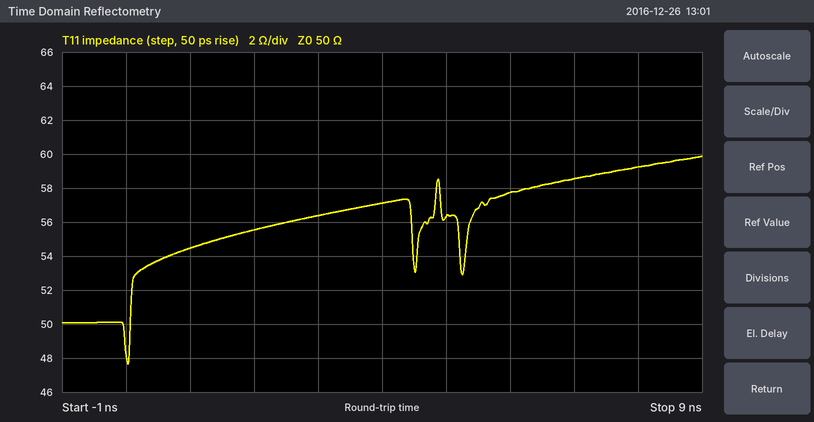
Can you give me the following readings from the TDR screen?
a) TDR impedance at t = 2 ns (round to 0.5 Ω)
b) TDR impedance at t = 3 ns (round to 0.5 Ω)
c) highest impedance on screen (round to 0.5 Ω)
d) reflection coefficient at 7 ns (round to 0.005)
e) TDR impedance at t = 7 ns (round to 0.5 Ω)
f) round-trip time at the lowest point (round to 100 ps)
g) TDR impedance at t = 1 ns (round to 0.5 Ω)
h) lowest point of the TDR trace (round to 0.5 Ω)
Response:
55.5 Ω
56.5 Ω
60.0 Ω
+0.080
58.5 Ω
0.0 ns
54.5 Ω
47.5 Ω
